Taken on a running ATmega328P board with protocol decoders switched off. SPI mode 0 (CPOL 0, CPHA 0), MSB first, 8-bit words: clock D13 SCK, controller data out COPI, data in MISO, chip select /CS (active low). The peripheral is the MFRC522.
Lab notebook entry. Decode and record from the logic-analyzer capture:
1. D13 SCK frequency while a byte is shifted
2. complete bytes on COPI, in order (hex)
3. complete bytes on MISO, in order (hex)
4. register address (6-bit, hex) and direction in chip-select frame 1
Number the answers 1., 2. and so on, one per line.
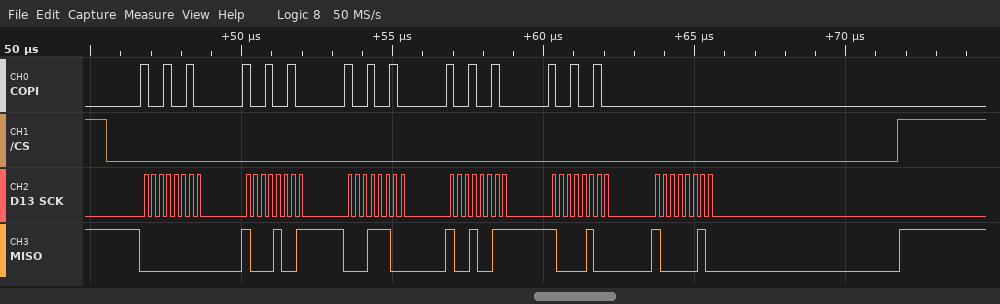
1. 4 MHz
2. 0x92 0x92 0x92 0x92 0x92 0x00
3. 0x00 0x89 0x1C 0x93 0x84 0x82
4. 0x09 read
